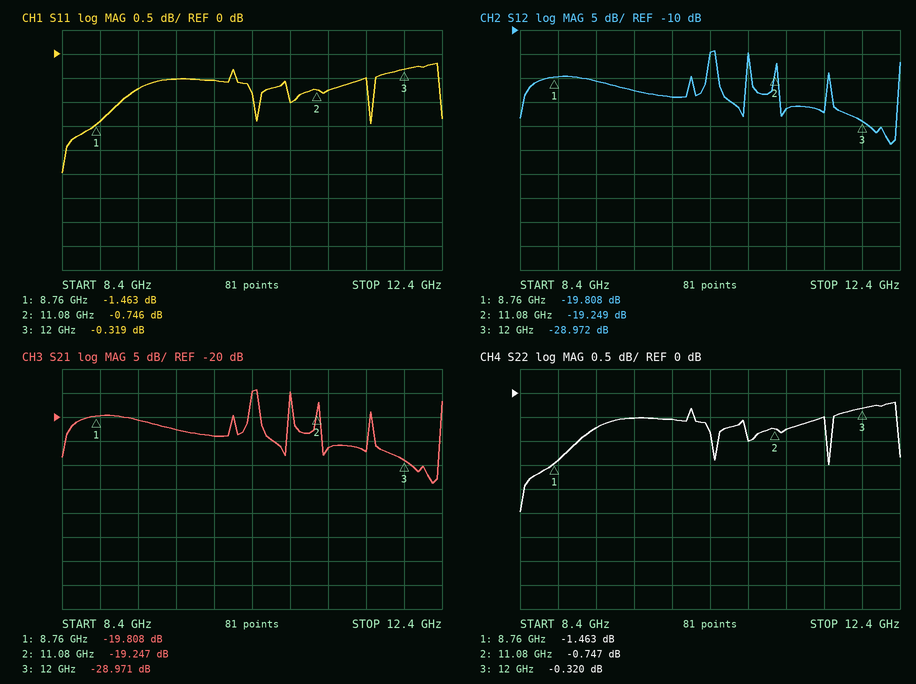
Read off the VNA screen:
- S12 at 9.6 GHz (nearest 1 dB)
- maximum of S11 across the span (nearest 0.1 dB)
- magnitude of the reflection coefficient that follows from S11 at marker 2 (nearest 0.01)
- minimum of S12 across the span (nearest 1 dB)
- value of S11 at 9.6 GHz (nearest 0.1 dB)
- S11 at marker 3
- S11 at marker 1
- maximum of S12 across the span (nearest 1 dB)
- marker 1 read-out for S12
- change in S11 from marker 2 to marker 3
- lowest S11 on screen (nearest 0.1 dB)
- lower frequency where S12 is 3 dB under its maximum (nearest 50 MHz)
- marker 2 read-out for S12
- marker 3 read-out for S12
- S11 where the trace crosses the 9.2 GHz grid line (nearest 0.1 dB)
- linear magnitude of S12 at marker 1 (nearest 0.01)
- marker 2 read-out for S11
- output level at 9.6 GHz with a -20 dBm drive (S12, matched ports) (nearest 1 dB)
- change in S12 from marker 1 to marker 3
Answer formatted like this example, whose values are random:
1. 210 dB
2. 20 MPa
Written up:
1. -23 dB
2. -0.2 dB
3. 0.92
4. -34 dB
5. -0.5 dB
6. -0.319 dB
7. -1.463 dB
8. -14 dB
9. -19.808 dB
10. 0.427 dB
11. -2.5 dB
12. 10.40 GHz
13. -19.249 dB
14. -28.972 dB
15. -0.7 dB
16. 0.10
17. -0.746 dB
18. -43 dBm
19. -9.164 dB
